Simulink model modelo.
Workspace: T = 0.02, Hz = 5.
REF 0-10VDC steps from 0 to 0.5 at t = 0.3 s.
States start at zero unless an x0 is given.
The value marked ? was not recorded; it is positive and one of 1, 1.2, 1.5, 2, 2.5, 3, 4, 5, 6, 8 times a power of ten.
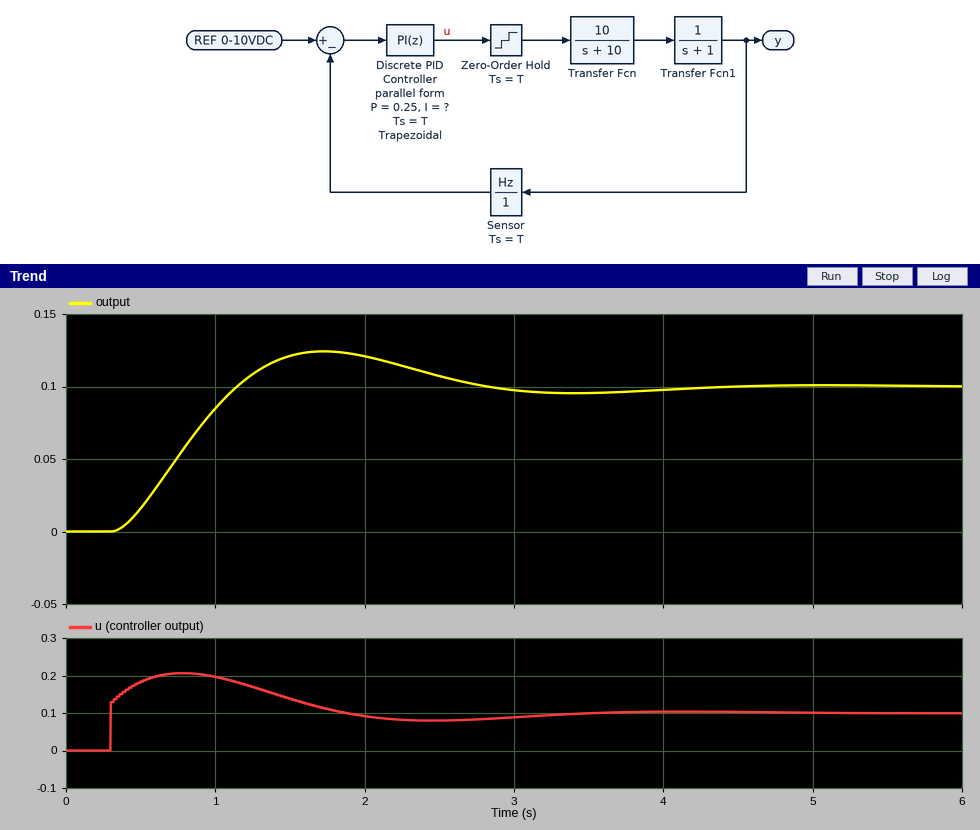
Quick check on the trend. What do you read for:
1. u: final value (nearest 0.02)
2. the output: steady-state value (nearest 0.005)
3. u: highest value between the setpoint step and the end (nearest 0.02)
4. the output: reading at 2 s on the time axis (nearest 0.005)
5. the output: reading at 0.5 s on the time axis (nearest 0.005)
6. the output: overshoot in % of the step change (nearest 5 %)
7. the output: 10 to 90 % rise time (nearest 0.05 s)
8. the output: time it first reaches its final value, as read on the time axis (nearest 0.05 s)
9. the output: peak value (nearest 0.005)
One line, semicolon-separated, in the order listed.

0.10; 0.100; 0.20; 0.120; 0.015; 25 %; 0.60 s; 1.15 s; 0.125
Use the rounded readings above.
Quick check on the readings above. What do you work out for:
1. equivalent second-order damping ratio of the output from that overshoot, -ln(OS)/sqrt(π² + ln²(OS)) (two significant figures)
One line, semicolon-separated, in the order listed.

0.40
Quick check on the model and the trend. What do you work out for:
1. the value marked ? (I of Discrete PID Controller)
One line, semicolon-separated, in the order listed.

0.8
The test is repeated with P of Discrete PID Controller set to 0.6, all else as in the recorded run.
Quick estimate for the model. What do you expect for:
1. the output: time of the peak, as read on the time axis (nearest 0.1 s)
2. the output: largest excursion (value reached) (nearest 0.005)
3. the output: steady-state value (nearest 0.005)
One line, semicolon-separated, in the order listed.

1.3 s; 0.105; 0.100
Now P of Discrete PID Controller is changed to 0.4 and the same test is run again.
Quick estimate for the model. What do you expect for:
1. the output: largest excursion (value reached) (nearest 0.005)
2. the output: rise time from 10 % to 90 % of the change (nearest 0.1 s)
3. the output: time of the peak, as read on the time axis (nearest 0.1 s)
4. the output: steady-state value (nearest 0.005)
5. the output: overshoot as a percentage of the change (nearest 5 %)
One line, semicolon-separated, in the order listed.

0.115; 0.5 s; 1.6 s; 0.100; 15 %
